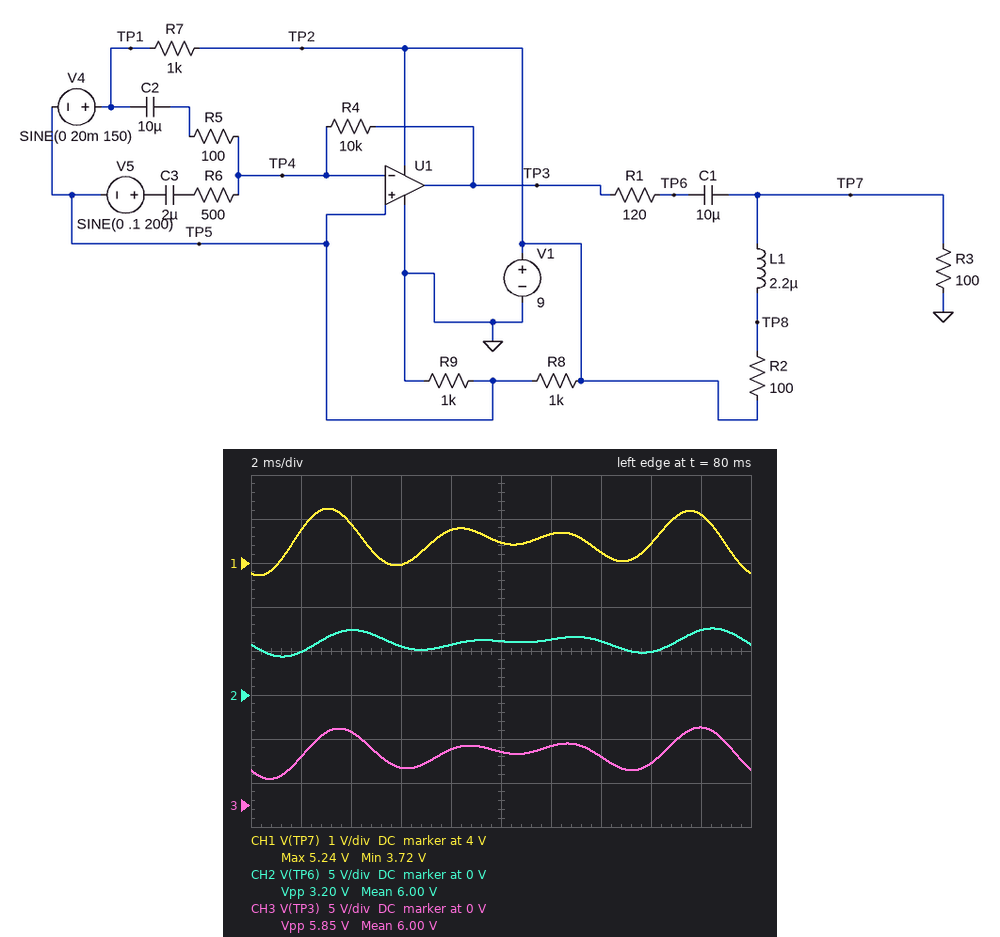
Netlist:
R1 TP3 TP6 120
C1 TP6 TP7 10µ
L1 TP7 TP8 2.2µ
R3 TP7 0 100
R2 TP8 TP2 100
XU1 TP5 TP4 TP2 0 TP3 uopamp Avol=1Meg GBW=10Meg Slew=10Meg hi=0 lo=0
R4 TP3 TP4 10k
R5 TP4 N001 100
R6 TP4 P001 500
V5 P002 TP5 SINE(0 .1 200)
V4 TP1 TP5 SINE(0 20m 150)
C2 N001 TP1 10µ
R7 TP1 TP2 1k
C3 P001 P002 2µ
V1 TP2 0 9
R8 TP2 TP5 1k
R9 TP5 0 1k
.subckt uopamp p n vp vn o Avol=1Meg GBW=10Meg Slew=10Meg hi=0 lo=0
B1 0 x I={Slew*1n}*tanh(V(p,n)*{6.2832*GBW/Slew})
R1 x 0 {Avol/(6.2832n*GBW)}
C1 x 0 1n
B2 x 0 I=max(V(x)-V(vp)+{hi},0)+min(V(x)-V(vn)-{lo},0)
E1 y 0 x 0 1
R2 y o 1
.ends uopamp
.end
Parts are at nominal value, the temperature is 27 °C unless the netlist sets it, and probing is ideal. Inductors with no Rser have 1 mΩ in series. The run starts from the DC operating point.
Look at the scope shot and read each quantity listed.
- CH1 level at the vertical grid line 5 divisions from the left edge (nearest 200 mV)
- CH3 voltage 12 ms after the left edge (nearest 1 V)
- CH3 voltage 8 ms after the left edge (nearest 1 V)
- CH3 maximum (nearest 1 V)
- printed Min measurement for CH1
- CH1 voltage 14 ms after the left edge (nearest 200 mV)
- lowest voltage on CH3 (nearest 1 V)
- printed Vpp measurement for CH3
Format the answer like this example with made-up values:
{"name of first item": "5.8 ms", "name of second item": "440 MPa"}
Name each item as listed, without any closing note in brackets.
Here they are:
{"CH1 level at the vertical grid line 5 divisions from the left edge": "4.4 V", "CH3 voltage 12 ms after the left edge": "7 V", "CH3 voltage 8 ms after the left edge": "6 V", "CH3 maximum": "9 V", "printed Min measurement for CH1": "3.72 V", "CH1 voltage 14 ms after the left edge": "4.2 V", "lowest voltage on CH3": "3 V", "printed Vpp measurement for CH3": "5.85 V"}
